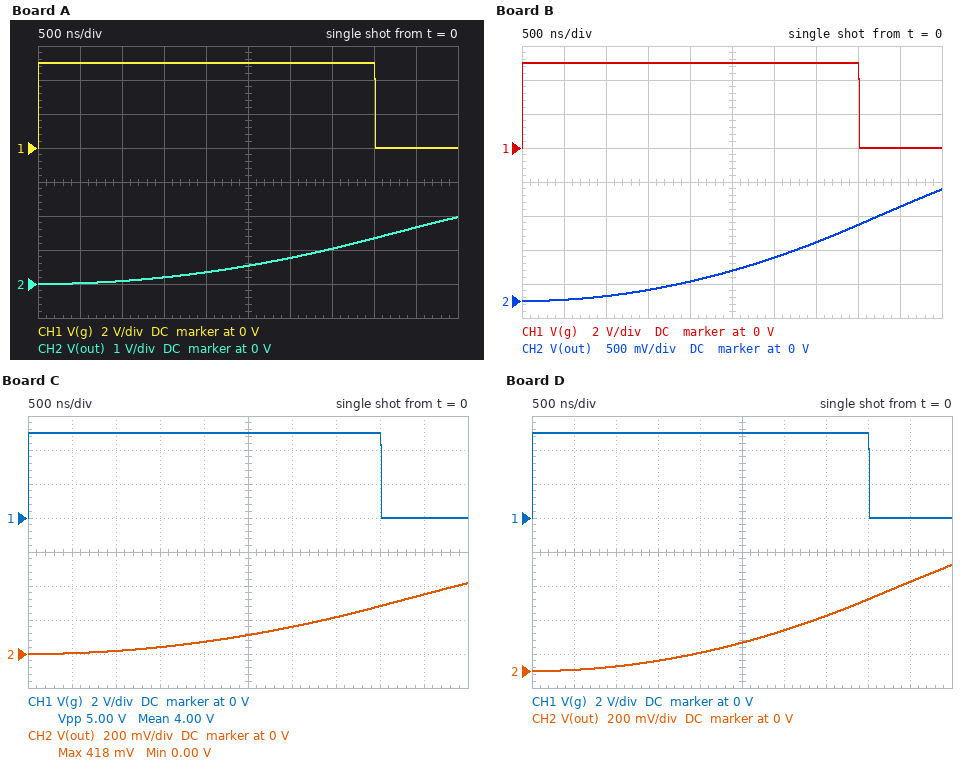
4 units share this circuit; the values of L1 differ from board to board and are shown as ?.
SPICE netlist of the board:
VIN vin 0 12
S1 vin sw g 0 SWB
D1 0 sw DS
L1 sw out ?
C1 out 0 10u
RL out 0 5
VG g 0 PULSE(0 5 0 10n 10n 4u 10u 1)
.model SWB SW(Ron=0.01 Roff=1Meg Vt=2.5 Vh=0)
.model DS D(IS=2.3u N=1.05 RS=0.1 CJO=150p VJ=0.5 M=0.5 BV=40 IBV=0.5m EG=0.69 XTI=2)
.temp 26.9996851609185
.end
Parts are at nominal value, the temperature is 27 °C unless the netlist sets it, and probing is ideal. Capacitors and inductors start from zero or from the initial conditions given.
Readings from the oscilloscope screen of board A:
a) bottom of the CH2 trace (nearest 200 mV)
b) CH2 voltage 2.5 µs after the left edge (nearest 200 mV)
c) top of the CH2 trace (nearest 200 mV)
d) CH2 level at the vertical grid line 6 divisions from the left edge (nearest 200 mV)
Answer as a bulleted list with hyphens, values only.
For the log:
- 0 V
- 600 mV
- 2.0 V
- 800 mV
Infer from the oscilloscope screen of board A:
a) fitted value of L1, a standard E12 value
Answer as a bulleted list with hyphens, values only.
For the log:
- 6.8 µH
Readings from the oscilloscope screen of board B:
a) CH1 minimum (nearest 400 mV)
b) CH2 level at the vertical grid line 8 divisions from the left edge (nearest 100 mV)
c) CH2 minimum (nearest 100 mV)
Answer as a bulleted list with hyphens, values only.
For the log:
- 0 V
- 1.1 V
- 0 V
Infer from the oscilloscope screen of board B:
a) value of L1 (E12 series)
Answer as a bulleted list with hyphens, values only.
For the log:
- 8.2 µH
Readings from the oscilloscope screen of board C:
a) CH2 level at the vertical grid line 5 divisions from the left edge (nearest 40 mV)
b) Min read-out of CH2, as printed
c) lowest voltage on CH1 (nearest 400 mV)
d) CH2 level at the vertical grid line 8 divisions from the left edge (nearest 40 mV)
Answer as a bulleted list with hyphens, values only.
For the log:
- 120 mV
- 0.00 V
- 0 V
- 280 mV
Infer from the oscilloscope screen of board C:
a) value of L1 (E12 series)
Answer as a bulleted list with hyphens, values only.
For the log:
- 33 µH
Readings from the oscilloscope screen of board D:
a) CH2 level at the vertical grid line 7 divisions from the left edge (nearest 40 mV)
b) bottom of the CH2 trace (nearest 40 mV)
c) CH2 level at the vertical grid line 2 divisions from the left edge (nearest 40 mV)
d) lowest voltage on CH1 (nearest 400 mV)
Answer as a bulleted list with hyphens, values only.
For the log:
- 320 mV
- 0 V
- 40 mV
- 0 V
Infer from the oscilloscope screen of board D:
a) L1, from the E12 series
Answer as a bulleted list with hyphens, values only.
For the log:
- 22 µH
